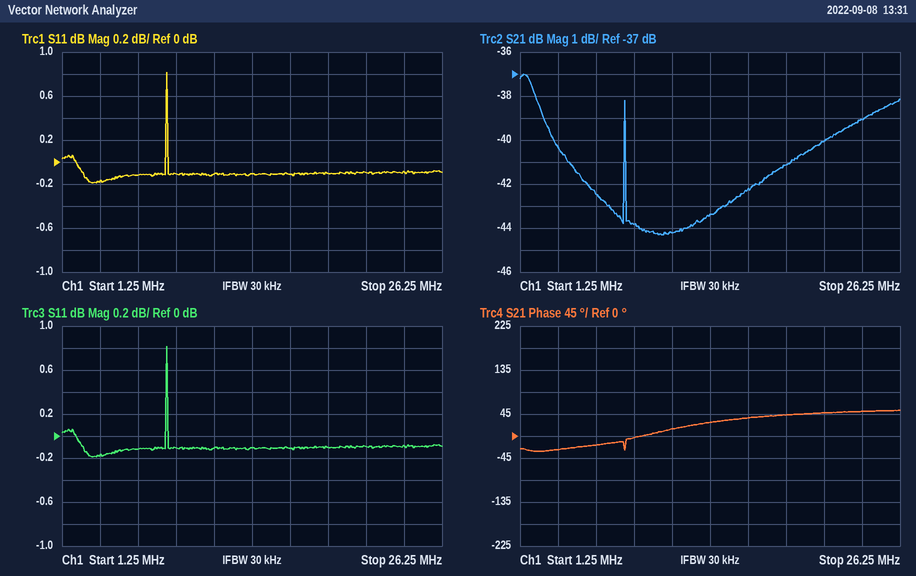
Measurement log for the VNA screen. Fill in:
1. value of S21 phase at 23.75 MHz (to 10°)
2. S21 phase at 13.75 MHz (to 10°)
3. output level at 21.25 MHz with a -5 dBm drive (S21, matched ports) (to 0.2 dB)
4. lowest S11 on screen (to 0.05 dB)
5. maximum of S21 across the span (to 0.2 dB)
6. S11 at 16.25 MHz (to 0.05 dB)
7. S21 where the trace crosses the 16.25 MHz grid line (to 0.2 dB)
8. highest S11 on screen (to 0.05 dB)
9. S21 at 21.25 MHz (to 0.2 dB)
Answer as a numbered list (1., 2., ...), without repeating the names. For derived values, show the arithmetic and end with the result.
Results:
1. 50°
2. 30°
3. -5 dBm + (-40.0 dB) = -45.0 dBm
4. -0.20 dB
5. -37.0 dB
6. -0.10 dB
7. -42.2 dB
8. 0.80 dB
9. -40.0 dB
